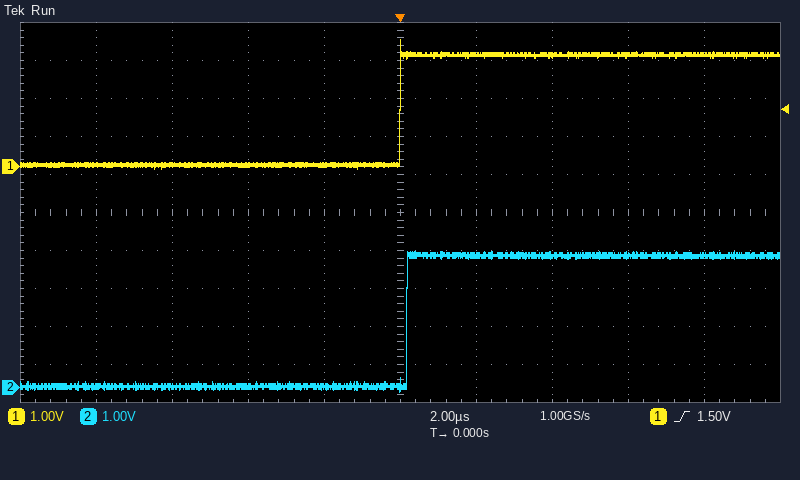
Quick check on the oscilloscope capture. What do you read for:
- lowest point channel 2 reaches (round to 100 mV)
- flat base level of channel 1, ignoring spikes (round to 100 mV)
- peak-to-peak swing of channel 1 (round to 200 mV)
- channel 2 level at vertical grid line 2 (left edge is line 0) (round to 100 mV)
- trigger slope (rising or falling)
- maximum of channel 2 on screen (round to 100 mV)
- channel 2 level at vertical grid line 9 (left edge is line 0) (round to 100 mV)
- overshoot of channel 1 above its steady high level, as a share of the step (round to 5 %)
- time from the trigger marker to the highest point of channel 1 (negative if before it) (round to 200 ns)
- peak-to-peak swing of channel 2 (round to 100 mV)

-100 mV
100 mV
3.4 V
0.0 V
rising
3.6 V
3.5 V
15 %
0.0 µs
3.7 V
